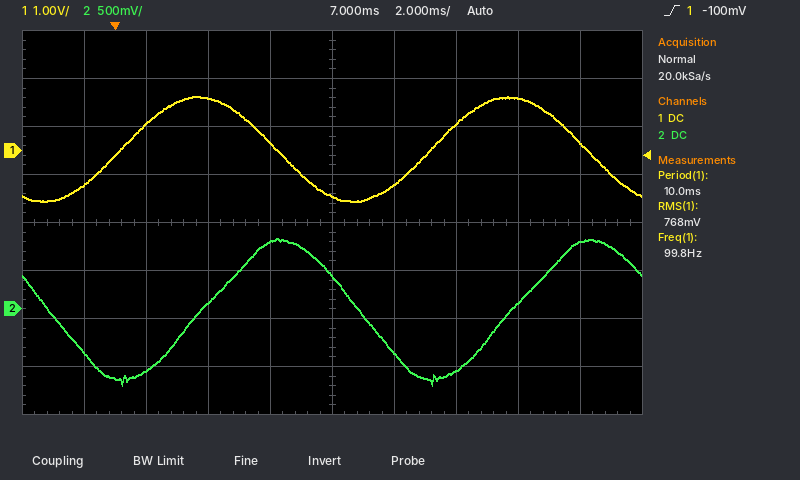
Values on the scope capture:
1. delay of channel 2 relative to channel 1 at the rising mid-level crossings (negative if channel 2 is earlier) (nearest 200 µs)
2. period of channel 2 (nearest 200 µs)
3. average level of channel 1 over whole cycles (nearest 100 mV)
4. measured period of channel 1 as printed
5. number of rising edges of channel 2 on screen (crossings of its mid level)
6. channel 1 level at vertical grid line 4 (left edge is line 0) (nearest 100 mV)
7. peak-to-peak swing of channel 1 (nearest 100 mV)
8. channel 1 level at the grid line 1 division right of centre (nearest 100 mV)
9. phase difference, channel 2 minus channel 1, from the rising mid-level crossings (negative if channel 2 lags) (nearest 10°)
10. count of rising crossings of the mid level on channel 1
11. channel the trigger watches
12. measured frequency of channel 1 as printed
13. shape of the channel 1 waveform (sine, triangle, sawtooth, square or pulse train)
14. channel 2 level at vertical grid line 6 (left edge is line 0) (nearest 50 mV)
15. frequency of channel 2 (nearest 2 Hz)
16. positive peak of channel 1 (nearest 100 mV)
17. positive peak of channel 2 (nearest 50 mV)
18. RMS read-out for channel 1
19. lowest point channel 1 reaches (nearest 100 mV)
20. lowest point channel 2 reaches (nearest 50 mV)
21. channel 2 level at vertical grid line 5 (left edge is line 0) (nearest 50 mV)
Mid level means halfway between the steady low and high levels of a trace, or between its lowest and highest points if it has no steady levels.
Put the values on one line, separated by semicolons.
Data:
+2.6 ms; 10.0 ms; 0.0 V; 10.0 ms; 2; 200 mV; 2.2 V; -700 mV; -90°; 2; channel 1; 99.8 Hz; sine; -450 mV; 100 Hz; 1.1 V; 750 mV; 768 mV; -1.1 V; -800 mV; 350 mV
